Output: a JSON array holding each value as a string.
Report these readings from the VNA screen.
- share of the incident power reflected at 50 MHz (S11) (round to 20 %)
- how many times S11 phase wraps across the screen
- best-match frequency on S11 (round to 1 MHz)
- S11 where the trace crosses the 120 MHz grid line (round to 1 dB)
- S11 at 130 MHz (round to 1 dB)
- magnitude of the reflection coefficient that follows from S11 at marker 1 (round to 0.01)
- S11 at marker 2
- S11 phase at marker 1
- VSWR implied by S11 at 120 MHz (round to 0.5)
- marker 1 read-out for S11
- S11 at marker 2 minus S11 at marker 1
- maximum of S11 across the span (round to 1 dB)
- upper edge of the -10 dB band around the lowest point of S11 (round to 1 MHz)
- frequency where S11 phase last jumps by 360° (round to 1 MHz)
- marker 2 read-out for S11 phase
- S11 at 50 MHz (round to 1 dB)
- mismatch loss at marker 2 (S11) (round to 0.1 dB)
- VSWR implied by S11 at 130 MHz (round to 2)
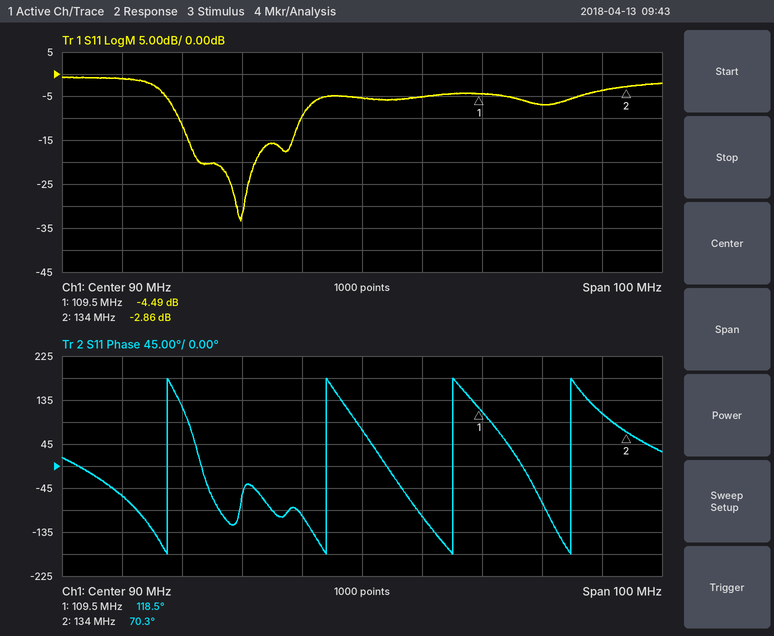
["80 %", "4", "70 MHz", "-7 dB", "-4 dB", "0.60", "-2.86 dB", "118.5°", "2.5", "-4.49 dB", "1.63 dB", "-1 dB", "80 MHz", "125 MHz", "70.3°", "-1 dB", "3.2 dB", "4"]
